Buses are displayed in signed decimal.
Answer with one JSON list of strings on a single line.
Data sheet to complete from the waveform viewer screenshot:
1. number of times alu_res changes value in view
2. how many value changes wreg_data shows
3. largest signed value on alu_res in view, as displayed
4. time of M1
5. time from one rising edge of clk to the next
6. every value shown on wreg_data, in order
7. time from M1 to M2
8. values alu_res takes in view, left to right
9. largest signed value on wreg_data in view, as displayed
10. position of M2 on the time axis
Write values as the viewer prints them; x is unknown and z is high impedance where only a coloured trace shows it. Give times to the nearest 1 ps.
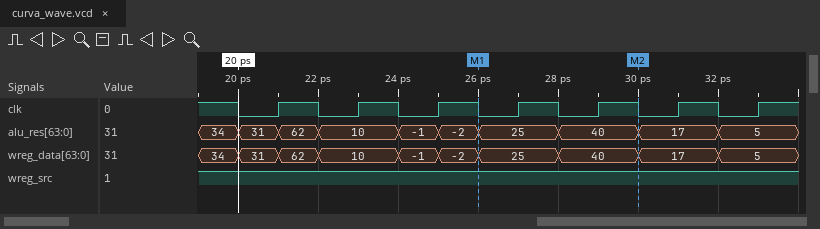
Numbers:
["9", "9", "62", "26 ps", "2 ps", "34, 31, 62, 10, -1, -2, 25, 40, 17, 5", "4 ps", "34, 31, 62, 10, -1, -2, 25, 40, 17, 5", "62", "30 ps"]
